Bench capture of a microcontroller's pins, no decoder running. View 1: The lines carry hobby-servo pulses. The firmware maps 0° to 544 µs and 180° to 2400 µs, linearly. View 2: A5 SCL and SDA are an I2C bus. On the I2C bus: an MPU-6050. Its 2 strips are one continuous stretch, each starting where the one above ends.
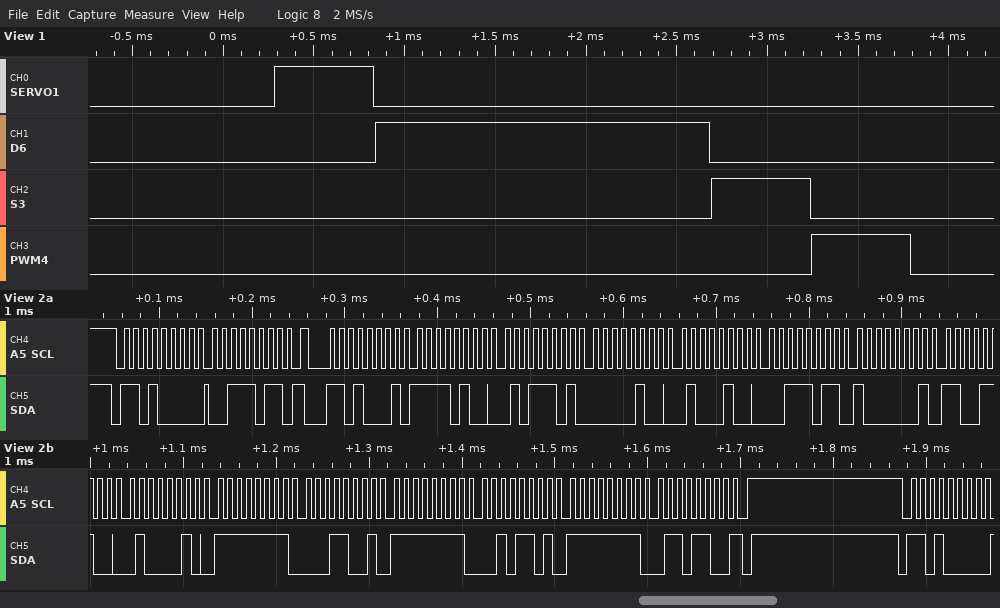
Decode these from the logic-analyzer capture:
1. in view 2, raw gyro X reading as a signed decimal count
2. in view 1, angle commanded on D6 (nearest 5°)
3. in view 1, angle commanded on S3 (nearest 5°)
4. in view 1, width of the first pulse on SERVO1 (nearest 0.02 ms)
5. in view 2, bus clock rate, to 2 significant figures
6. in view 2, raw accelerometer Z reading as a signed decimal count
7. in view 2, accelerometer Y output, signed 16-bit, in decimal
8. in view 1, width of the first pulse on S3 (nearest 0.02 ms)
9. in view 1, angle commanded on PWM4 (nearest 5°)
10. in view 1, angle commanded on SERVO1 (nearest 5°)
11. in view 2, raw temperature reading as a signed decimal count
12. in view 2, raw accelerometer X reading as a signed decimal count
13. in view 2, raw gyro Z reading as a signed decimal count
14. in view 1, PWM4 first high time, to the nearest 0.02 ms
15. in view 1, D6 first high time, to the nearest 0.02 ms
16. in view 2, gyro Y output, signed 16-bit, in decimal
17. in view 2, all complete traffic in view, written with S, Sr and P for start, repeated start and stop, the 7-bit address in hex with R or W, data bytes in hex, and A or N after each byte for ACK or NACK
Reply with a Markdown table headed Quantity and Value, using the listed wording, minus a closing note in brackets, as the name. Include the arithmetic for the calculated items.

| Quantity | Value |
|---|---|
| in view 2, raw gyro X reading as a signed decimal count | 0xFF19 = -231 |
| in view 1, angle commanded on D6 | 125° |
| in view 1, angle commanded on S3 | 0° |
| in view 1, width of the first pulse on SERVO1 | 0.54 ms |
| in view 2, bus clock rate, to 2 significant figures | 100 kHz |
| in view 2, raw accelerometer Z reading as a signed decimal count | 0x3B81 = 15233 |
| in view 2, accelerometer Y output, signed 16-bit, in decimal | 0x0444 = 1092 |
| in view 1, width of the first pulse on S3 | 0.54 ms |
| in view 1, angle commanded on PWM4 | 0° |
| in view 1, angle commanded on SERVO1 | 0° |
| in view 2, raw temperature reading as a signed decimal count | 0xCC42 = -13246 |
| in view 2, raw accelerometer X reading as a signed decimal count | 0xF45D = -2979 |
| in view 2, raw gyro Z reading as a signed decimal count | 0xFF6C = -148 |
| in view 1, PWM4 first high time, to the nearest 0.02 ms | 0.54 ms |
| in view 1, D6 first high time, to the nearest 0.02 ms | 1.84 ms |
| in view 2, gyro Y output, signed 16-bit, in decimal | 0xFF2D = -211 |
| in view 2, all complete traffic in view, written with S, Sr and P for start, repeated start and stop, the 7-bit address in hex with R or W, data bytes in hex, and A or N after each byte for ACK or NACK | S 68W A 3B A Sr 68R A F4 A 5D A 04 A 44 A 3B A 81 A CC A 42 A FF A 19 A FF A 2D A FF A 6C N P S 68W A |
